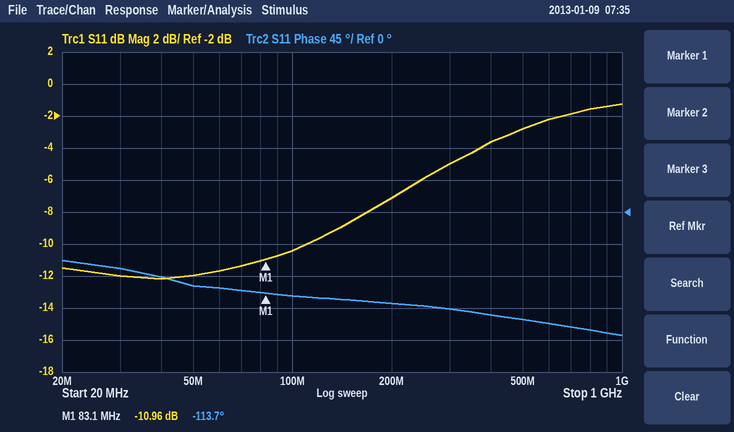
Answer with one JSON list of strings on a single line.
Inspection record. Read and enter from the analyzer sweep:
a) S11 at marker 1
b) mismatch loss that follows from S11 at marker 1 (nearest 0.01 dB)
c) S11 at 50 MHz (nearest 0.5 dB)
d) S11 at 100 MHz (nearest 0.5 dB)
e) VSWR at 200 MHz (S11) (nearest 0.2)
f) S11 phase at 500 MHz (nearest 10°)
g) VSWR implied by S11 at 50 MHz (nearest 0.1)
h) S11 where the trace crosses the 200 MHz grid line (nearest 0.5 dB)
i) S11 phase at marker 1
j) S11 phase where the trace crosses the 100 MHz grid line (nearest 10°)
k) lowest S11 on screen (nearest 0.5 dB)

["-10.96 dB", "0.36 dB", "-12.0 dB", "-10.5 dB", "2.6", "-150°", "1.7", "-7.0 dB", "-113.7°", "-120°", "-12.0 dB"]
